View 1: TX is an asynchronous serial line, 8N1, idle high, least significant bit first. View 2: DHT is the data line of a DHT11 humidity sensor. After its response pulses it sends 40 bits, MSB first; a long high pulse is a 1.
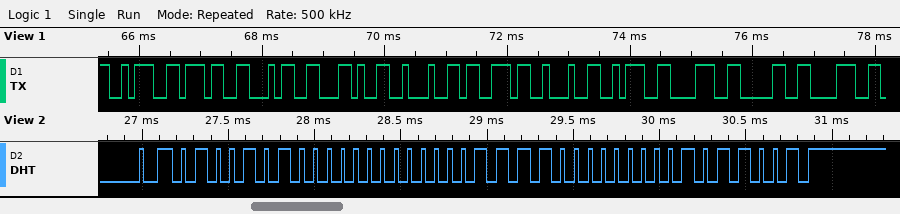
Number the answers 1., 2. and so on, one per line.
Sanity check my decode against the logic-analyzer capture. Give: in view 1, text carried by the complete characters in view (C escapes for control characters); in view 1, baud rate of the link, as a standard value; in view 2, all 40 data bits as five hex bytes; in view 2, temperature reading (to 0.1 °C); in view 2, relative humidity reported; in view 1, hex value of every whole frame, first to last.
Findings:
1. ":74,\"s\":808"
2. 9600 baud
3. 4A 00 0F 00 59
4. 15.0 °C
5. 74 %
6. 3A 37 34 2C 22 73 22 3A 38 30 38
